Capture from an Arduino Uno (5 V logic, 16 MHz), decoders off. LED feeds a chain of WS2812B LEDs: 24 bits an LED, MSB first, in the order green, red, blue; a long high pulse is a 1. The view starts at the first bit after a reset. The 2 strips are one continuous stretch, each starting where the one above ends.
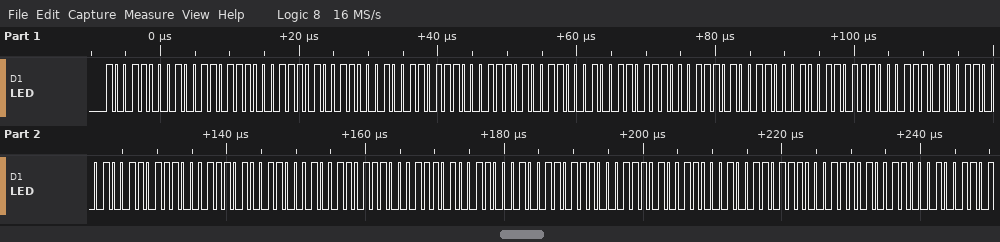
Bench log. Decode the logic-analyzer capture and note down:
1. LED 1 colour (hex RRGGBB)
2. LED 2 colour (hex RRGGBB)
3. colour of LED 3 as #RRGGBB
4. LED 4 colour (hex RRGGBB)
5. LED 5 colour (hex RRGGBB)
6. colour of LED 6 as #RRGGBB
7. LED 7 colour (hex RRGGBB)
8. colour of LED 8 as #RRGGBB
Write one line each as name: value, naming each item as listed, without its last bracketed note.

LED 1 colour: #9B988E
LED 2 colour: #9B988E
colour of LED 3 as #RRGGBB: #9B988E
LED 4 colour: #9B988E
LED 5 colour: #9B988E
colour of LED 6 as #RRGGBB: #9B988E
LED 7 colour: #9B988E
colour of LED 8 as #RRGGBB: #9B988E
